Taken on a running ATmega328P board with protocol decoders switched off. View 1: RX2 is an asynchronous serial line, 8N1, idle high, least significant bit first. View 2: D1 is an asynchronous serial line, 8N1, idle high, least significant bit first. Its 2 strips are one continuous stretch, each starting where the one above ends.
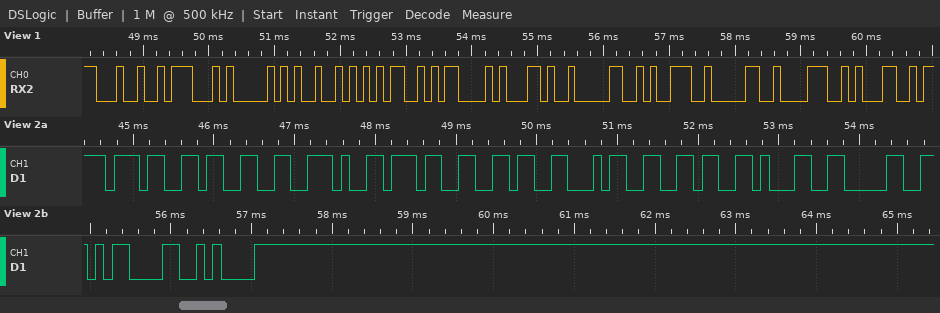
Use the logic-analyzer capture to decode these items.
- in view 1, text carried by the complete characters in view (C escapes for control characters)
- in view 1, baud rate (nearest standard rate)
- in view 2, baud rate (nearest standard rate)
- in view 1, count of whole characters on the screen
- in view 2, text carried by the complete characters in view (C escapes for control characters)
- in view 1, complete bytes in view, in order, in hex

"$GPRMC,09081"
9600 baud
9600 baud
12
"73.764610\r\n"
24 47 50 52 4D 43 2C 30 39 30 38 31
